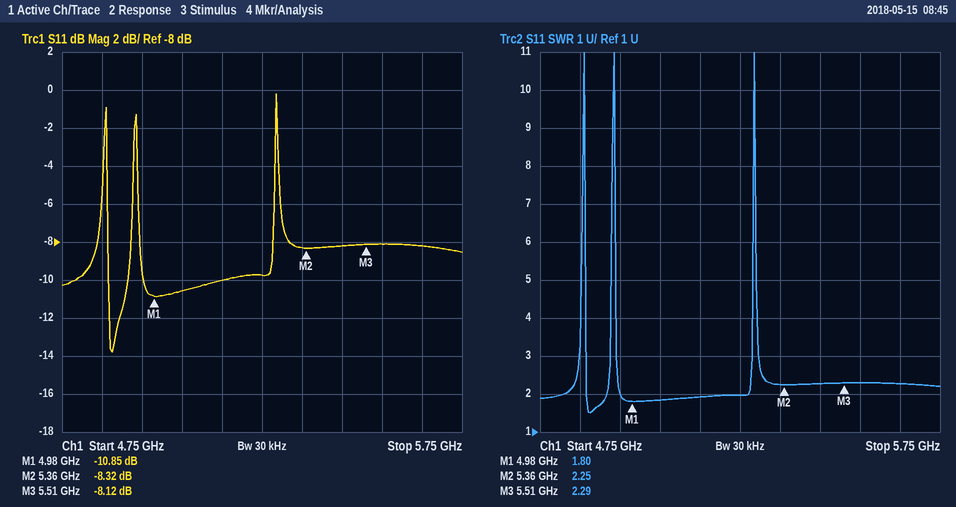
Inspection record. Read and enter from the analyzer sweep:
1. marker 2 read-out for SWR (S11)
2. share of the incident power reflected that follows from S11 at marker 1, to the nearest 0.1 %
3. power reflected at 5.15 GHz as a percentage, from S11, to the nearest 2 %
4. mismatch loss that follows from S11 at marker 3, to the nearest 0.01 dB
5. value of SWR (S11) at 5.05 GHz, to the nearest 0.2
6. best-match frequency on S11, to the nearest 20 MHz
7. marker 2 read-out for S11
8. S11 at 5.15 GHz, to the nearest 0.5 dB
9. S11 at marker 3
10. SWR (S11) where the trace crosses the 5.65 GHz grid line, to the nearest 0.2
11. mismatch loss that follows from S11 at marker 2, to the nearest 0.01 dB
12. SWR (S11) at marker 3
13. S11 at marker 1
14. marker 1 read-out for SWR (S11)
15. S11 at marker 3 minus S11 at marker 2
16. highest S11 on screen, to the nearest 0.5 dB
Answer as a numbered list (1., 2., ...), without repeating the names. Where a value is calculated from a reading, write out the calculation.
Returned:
1. 2.25
2. 10^(-10.85/10) ≈ 8.2 %
3. 10^(-10/10) ≈ 10 %
4. −10 log10(1 − 10^(-8.12/10)) ≈ 0.73 dB
5. 1.8
6. 4.88 GHz
7. -8.32 dB
8. -10.0 dB
9. -8.12 dB
10. 2.2
11. −10 log10(1 − 10^(-8.32/10)) ≈ 0.69 dB
12. 2.29
13. -10.85 dB
14. 1.80
15. -8.12 − (-8.32) = 0.20 dB
16. 0.0 dB
